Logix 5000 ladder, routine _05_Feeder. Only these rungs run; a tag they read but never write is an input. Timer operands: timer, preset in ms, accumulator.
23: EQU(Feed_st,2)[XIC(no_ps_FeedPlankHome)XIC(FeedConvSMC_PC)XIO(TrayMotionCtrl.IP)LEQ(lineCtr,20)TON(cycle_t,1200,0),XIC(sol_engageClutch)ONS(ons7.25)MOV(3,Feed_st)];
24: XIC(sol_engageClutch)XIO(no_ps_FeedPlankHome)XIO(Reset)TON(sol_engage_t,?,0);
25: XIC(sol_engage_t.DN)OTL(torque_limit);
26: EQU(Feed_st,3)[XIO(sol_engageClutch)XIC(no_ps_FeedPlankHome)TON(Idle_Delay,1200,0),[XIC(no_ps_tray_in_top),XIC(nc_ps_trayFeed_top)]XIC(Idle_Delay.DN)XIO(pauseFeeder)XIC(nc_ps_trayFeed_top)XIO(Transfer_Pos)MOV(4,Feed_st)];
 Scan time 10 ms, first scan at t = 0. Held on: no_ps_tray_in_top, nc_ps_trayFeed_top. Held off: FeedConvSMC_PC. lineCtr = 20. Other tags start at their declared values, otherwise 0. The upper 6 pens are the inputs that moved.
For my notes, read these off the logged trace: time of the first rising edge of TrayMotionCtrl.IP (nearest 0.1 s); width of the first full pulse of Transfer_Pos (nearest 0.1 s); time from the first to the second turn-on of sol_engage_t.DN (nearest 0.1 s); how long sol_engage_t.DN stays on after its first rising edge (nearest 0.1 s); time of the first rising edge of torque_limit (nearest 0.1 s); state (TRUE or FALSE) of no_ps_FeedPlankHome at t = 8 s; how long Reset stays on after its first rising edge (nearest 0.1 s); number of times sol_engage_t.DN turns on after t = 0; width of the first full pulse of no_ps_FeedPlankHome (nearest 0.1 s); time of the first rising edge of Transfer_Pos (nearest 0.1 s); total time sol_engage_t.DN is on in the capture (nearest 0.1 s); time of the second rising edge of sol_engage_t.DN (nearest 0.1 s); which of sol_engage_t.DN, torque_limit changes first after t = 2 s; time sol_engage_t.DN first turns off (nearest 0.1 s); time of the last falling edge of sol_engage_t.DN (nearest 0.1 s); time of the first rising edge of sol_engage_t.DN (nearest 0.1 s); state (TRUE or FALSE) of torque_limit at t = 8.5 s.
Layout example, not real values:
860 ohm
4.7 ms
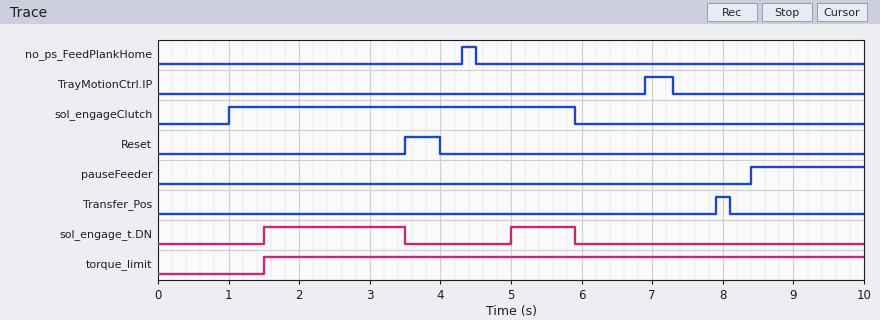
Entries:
6.9 s
0.2 s
3.5 s
2.0 s
1.5 s
FALSE
0.5 s
2
0.2 s
7.9 s
2.9 s
5.0 s
sol_engage_t.DN
3.5 s
5.9 s
1.5 s
TRUE
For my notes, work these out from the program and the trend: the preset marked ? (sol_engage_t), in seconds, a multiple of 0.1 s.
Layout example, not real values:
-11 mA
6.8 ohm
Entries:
0.5 s
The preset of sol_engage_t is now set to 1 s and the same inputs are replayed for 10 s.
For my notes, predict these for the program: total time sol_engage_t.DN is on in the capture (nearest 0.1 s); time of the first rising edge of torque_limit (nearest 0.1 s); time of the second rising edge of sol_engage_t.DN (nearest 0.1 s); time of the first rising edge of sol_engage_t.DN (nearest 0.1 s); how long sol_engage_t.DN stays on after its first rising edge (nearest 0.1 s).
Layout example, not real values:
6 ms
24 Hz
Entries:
1.9 s
2.0 s
5.5 s
2.0 s
1.5 s
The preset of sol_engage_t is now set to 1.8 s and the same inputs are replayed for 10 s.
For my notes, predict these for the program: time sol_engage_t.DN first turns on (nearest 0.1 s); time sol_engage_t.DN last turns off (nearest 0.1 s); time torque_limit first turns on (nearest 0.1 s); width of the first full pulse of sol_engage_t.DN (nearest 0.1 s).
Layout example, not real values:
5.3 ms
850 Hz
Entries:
2.8 s
3.5 s
2.8 s
0.7 s
